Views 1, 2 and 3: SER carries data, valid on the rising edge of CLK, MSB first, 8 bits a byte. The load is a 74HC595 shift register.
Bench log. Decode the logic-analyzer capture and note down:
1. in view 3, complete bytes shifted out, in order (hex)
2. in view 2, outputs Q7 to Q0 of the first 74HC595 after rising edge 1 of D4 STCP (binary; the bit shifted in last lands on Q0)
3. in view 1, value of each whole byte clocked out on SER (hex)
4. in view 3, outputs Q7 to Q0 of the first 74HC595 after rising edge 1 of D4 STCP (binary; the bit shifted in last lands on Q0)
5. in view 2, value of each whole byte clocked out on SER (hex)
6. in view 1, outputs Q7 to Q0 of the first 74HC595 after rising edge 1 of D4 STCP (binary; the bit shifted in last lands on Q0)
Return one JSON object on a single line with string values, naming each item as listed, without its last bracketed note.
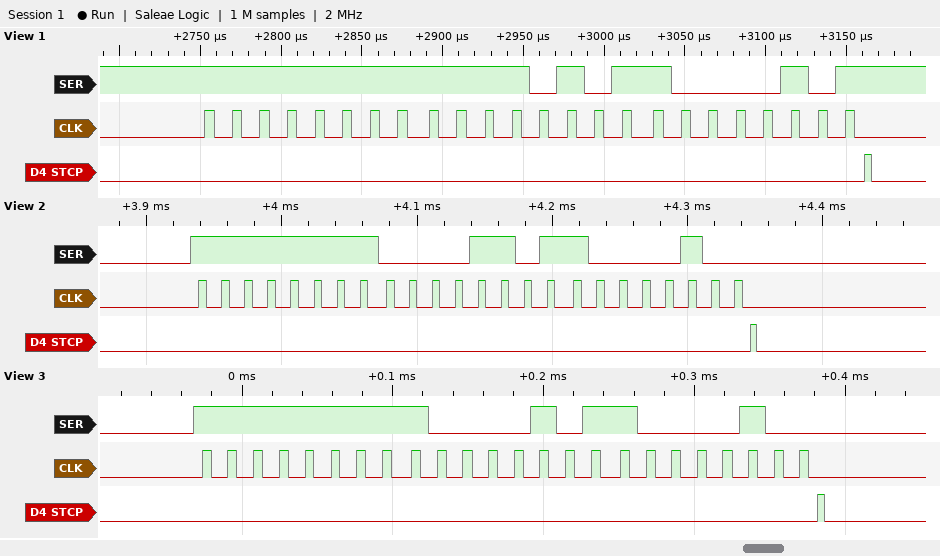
{"in view 3, complete bytes shifted out, in order": "0xFF 0x85 0x84", "in view 2, outputs Q7 to Q0 of the first 74HC595 after rising edge 1 of D4 STCP": "10000100", "in view 1, value of each whole byte clocked out on SER": "FF F5 85", "in view 3, outputs Q7 to Q0 of the first 74HC595 after rising edge 1 of D4 STCP": "10000100", "in view 2, value of each whole byte clocked out on SER": "0xFF 0x0D 0x84", "in view 1, outputs Q7 to Q0 of the first 74HC595 after rising edge 1 of D4 STCP": "10000101"}
